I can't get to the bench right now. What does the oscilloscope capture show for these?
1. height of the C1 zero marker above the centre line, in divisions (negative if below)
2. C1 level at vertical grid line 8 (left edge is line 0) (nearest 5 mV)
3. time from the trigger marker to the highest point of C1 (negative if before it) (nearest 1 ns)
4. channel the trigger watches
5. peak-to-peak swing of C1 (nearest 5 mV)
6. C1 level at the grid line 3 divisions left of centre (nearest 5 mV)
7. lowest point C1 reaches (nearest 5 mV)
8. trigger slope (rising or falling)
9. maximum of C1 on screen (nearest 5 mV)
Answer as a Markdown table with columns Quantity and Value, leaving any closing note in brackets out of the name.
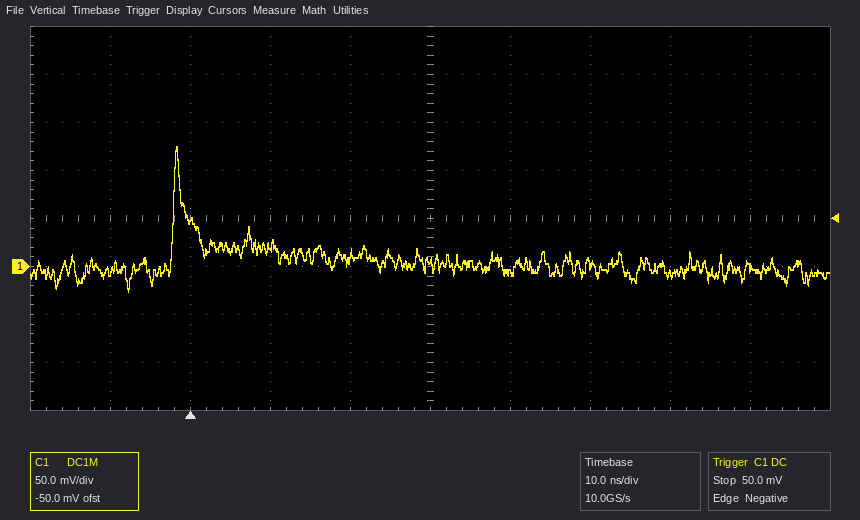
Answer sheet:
| Quantity | Value |
|---|---|
| height of the C1 zero marker above the centre line, in divisions | -1.0 div |
| C1 level at vertical grid line 8 (left edge is line 0) | -10 mV |
| time from the trigger marker to the highest point of C1 (negative if before it) | -2 ns |
| channel the trigger watches | C1 |
| peak-to-peak swing of C1 | 150 mV |
| C1 level at the grid line 3 divisions left of centre | 50 mV |
| lowest point C1 reaches | -25 mV |
| trigger slope | falling |
| maximum of C1 on screen | 125 mV |
